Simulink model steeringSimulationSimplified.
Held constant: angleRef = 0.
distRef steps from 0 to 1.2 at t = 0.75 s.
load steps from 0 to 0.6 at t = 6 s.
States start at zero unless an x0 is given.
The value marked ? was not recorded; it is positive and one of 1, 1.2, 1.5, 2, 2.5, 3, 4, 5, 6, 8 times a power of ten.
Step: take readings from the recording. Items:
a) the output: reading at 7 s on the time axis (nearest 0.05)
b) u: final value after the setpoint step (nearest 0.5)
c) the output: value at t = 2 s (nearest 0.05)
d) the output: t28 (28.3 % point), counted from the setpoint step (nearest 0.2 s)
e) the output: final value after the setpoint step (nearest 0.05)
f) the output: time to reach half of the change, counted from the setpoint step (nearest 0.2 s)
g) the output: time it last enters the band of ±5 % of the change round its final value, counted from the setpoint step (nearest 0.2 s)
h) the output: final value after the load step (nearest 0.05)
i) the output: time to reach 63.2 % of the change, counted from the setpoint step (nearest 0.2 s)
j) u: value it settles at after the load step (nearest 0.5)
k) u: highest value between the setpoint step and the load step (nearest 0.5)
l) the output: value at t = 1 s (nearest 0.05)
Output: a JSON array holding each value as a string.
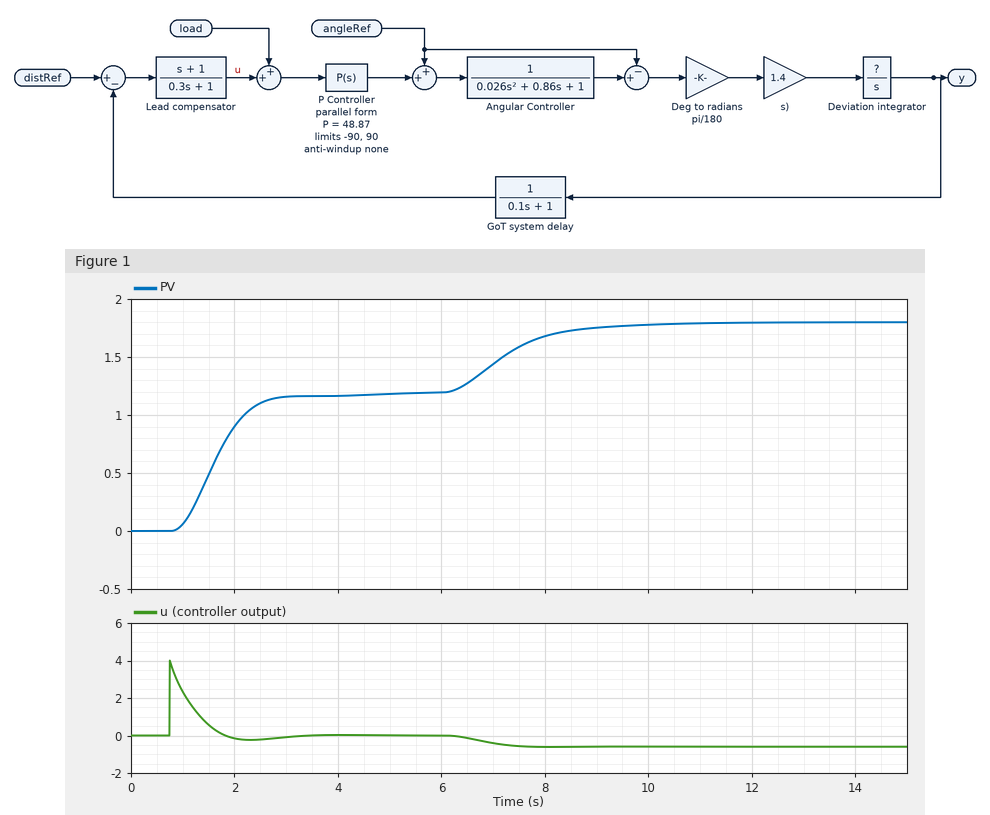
["1.45", "0.0", "0.90", "0.6 s", "1.20", "0.8 s", "2.0 s", "1.80", "1.0 s", "-0.5", "4.0", "0.05"]
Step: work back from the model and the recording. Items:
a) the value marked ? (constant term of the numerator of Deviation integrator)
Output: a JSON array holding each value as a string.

["1"]
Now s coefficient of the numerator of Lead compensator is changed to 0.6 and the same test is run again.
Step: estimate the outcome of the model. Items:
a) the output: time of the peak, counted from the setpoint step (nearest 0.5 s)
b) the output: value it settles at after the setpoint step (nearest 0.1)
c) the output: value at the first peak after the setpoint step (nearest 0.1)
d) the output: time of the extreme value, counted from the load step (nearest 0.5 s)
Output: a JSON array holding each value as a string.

["2.5 s", "1.2", "1.3", "3.0 s"]
